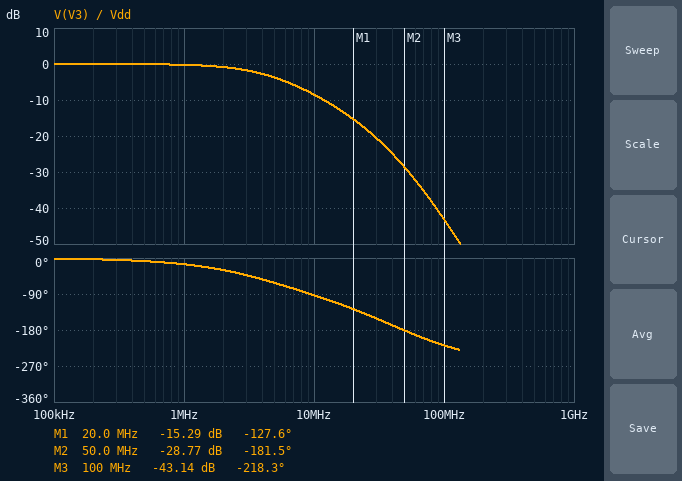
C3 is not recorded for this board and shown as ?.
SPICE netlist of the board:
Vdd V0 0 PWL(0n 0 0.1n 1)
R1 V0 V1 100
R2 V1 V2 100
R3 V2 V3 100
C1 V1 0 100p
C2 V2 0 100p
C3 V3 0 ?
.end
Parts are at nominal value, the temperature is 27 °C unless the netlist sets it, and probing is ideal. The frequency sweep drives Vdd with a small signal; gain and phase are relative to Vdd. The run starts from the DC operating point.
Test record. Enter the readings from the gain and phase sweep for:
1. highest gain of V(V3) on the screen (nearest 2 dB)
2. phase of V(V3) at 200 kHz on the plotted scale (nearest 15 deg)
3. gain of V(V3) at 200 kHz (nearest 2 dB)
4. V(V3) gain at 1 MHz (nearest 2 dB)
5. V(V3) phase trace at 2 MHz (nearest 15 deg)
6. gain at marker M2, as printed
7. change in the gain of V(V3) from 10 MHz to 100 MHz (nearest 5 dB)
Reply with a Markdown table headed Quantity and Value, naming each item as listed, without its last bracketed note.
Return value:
| Quantity | Value |
|---|---|
| highest gain of V(V3) on the screen | 0 dB |
| phase of V(V3) at 200 kHz on the plotted scale | 0 deg |
| gain of V(V3) at 200 kHz | 0 dB |
| V(V3) gain at 1 MHz | 0 dB |
| V(V3) phase trace at 2 MHz | -30 deg |
| gain at marker M2, as printed | -28.77 dB |
| change in the gain of V(V3) from 10 MHz to 100 MHz | -35 dB |
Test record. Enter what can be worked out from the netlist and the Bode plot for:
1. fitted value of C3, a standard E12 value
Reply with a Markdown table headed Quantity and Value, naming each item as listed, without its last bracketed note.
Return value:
| Quantity | Value |
|---|---|
| fitted value of C3, a standard E12 value | 47 pF |
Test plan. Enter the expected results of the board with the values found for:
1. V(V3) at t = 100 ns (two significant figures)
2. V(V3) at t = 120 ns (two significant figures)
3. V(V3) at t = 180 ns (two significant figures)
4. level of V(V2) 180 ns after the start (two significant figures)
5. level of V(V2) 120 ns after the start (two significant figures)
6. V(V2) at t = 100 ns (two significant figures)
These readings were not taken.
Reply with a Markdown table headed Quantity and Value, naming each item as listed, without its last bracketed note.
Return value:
| Quantity | Value |
|---|---|
| V(V3) at t = 100 ns | 920 mV |
| V(V3) at t = 120 ns | 950 mV |
| V(V3) at t = 180 ns | 990 mV |
| level of V(V2) 180 ns after the start | 990 mV |
| level of V(V2) 120 ns after the start | 960 mV |
| V(V2) at t = 100 ns | 930 mV |
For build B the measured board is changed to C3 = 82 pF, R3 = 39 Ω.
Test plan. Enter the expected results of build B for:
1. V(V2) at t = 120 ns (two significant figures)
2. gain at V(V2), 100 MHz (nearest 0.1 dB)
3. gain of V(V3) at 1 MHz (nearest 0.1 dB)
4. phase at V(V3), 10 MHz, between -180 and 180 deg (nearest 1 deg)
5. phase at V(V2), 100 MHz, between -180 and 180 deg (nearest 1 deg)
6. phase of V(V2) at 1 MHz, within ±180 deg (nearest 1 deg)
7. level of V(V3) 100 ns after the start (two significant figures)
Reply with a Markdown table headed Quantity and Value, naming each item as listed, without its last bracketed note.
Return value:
| Quantity | Value |
|---|---|
| V(V2) at t = 120 ns | 930 mV |
| gain at V(V2), 100 MHz | -34.5 dB |
| gain of V(V3) at 1 MHz | -0.3 dB |
| phase at V(V3), 10 MHz, between -180 and 180 deg | -92 deg |
| phase at V(V2), 100 MHz, between -180 and 180 deg | -140 deg |
| phase of V(V2) at 1 MHz, within ±180 deg | -16 deg |
| level of V(V3) 100 ns after the start | 880 mV |
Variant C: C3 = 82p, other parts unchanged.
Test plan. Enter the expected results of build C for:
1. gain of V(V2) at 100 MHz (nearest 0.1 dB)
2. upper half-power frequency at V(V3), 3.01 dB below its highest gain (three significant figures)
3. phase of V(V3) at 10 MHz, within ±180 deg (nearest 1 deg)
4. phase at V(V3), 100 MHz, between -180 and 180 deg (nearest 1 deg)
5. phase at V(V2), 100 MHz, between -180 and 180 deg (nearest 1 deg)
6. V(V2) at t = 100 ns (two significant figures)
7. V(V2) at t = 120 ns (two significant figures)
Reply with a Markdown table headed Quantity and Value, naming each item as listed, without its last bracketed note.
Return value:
| Quantity | Value |
|---|---|
| gain of V(V2) at 100 MHz | -33.1 dB |
| upper half-power frequency at V(V3), 3.01 dB below its highest gain | 3.42 MHz |
| phase of V(V3) at 10 MHz, within ±180 deg | -102 deg |
| phase at V(V3), 100 MHz, between -180 and 180 deg | 135 deg |
| phase at V(V2), 100 MHz, between -180 and 180 deg | -146 deg |
| V(V2) at t = 100 ns | 890 mV |
| V(V2) at t = 120 ns | 930 mV |
